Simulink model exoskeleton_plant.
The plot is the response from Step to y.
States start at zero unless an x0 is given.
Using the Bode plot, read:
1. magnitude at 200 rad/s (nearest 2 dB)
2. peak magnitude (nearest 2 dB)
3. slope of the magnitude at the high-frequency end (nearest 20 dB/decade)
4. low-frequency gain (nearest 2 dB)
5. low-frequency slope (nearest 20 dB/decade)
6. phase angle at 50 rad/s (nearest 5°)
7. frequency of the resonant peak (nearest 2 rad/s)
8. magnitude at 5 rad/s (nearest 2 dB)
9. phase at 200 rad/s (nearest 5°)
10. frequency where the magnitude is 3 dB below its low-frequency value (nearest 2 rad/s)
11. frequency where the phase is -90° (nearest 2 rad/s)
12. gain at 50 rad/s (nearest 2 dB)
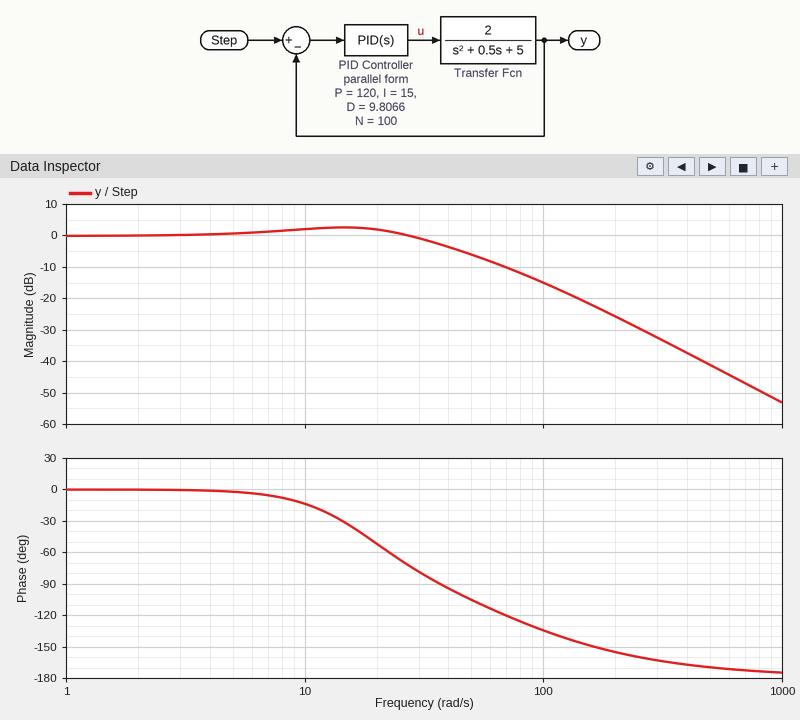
-26 dB
2 dB
-40 dB/decade
0 dB
0 dB/decade
-105°
14 rad/s
0 dB
-155°
38 rad/s
36 rad/s
-6 dB
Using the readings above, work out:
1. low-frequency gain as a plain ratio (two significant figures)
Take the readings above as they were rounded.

1.0
